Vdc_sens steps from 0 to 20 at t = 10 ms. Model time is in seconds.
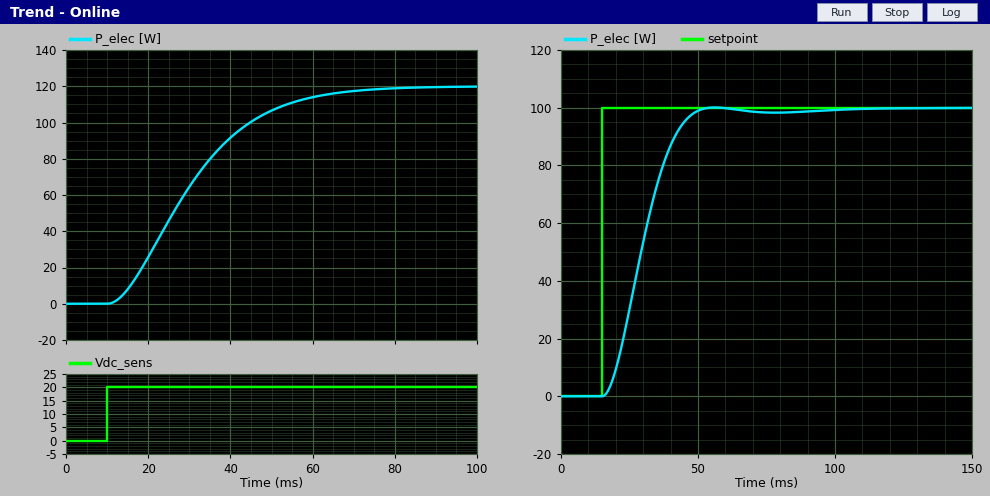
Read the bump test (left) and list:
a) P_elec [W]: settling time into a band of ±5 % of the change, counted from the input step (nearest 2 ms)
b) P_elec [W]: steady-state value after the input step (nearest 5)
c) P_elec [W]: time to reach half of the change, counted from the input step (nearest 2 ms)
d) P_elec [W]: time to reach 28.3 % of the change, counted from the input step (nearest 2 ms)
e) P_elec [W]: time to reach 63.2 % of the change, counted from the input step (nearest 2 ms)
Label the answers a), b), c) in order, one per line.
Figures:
a) 50 ms
b) 120
c) 18 ms
d) 12 ms
e) 24 ms
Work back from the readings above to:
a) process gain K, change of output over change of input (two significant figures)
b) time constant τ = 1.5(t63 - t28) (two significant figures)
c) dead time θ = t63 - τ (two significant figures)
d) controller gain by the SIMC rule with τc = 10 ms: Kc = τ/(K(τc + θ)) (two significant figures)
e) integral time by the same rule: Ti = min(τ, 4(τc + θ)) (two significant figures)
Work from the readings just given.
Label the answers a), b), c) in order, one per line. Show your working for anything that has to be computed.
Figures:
a) (120 - 0) / 20 = 6.0
b) 1.5 × (24 - 12) = 18 ms
c) 24 - 18 = 6.0 ms
d) 18 / (6 × (10 + 6)) = 0.19
e) min(18, 4 × (10 + 6)) = 18 ms
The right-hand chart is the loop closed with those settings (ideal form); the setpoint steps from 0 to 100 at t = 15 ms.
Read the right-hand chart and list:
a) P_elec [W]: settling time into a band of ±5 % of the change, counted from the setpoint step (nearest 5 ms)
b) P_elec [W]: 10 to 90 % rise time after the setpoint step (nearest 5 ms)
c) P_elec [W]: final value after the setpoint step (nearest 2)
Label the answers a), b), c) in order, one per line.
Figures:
a) 30 ms
b) 20 ms
c) 100
